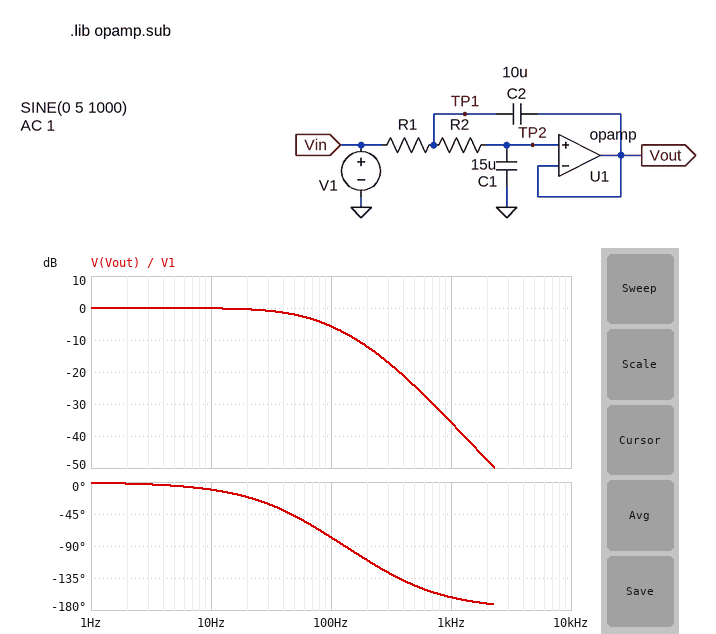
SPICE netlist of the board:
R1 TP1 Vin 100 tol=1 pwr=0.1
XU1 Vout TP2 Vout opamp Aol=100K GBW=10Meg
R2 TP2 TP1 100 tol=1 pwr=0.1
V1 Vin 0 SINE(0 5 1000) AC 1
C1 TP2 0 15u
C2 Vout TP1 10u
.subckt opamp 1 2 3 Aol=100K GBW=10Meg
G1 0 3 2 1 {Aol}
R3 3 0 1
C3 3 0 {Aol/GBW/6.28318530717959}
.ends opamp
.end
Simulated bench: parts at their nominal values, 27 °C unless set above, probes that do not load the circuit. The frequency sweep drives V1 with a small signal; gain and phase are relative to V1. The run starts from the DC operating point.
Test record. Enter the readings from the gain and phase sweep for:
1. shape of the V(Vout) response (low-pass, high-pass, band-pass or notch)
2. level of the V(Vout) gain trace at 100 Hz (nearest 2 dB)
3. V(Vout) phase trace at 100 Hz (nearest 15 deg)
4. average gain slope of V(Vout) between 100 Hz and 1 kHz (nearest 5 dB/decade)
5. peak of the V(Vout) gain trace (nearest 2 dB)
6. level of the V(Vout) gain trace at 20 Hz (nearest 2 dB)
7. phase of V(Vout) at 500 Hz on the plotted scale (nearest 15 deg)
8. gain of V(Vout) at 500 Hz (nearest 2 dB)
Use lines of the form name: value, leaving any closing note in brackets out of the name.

shape of the V(Vout) response: low-pass
level of the V(Vout) gain trace at 100 Hz: -6 dB
V(Vout) phase trace at 100 Hz: -75 deg
average gain slope of V(Vout) between 100 Hz and 1 kHz: -30 dB/decade
peak of the V(Vout) gain trace: 0 dB
level of the V(Vout) gain trace at 20 Hz: 0 dB
phase of V(Vout) at 500 Hz on the plotted scale: -150 deg
gain of V(Vout) at 500 Hz: -24 dB
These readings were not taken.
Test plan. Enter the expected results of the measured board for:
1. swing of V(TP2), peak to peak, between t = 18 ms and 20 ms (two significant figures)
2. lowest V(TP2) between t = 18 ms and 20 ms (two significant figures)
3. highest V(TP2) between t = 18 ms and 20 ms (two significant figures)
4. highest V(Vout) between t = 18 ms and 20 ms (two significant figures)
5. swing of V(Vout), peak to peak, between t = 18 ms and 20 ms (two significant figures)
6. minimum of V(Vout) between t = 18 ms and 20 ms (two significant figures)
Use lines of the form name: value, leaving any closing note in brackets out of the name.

swing of V(TP2), peak to peak, between t = 18 ms and 20 ms: 160 mV
lowest V(TP2) between t = 18 ms and 20 ms: -82 mV
highest V(TP2) between t = 18 ms and 20 ms: 82 mV
highest V(Vout) between t = 18 ms and 20 ms: 82 mV
swing of V(Vout), peak to peak, between t = 18 ms and 20 ms: 160 mV
minimum of V(Vout) between t = 18 ms and 20 ms: -82 mV
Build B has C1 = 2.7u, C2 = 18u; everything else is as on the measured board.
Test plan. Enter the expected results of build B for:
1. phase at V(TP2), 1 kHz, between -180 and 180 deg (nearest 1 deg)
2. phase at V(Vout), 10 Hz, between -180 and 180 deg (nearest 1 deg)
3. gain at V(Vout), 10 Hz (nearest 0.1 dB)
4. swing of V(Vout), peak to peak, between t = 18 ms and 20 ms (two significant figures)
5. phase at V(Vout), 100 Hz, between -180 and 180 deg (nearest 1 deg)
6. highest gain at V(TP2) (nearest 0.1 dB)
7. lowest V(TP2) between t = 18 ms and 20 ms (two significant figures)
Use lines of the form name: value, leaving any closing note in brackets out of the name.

phase at V(TP2), 1 kHz, between -180 and 180 deg: -169 deg
phase at V(Vout), 10 Hz, between -180 and 180 deg: -2 deg
gain at V(Vout), 10 Hz: 0 dB
swing of V(Vout), peak to peak, between t = 18 ms and 20 ms: 540 mV
phase at V(Vout), 100 Hz, between -180 and 180 deg: -23 deg
highest gain at V(TP2): 2.9 dB
lowest V(TP2) between t = 18 ms and 20 ms: -270 mV
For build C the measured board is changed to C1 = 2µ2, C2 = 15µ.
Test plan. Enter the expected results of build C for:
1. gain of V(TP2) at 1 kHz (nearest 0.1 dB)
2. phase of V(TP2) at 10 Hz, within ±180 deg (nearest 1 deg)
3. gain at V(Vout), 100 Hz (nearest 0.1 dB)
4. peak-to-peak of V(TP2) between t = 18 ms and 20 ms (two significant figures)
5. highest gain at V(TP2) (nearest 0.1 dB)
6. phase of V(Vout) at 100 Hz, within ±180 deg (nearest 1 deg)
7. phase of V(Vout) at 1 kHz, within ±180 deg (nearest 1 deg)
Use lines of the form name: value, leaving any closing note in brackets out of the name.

gain of V(TP2) at 1 kHz: -21.8 dB
phase of V(TP2) at 10 Hz, within ±180 deg: -2 deg
gain at V(Vout), 100 Hz: 0.8 dB
peak-to-peak of V(TP2) between t = 18 ms and 20 ms: 810 mV
highest gain at V(TP2): 3.0 dB
phase of V(Vout) at 100 Hz, within ±180 deg: -18 deg
phase of V(Vout) at 1 kHz, within ±180 deg: -167 deg
